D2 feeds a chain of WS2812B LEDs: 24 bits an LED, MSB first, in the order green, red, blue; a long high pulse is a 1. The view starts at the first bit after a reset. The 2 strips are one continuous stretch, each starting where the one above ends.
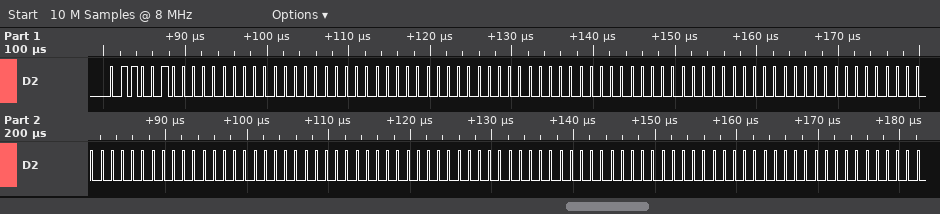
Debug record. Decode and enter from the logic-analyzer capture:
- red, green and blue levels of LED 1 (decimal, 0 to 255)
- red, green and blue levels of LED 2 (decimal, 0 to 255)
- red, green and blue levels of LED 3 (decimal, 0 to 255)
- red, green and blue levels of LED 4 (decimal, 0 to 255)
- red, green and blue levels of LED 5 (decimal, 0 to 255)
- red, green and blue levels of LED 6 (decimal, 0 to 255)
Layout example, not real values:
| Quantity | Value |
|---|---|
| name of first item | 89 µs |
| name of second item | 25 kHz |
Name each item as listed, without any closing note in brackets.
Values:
| Quantity | Value |
|---|---|
| red, green and blue levels of LED 1 | 0, 100, 0 |
| red, green and blue levels of LED 2 | 0, 0, 0 |
| red, green and blue levels of LED 3 | 0, 0, 0 |
| red, green and blue levels of LED 4 | 0, 0, 0 |
| red, green and blue levels of LED 5 | 0, 0, 0 |
| red, green and blue levels of LED 6 | 0, 0, 0 |
